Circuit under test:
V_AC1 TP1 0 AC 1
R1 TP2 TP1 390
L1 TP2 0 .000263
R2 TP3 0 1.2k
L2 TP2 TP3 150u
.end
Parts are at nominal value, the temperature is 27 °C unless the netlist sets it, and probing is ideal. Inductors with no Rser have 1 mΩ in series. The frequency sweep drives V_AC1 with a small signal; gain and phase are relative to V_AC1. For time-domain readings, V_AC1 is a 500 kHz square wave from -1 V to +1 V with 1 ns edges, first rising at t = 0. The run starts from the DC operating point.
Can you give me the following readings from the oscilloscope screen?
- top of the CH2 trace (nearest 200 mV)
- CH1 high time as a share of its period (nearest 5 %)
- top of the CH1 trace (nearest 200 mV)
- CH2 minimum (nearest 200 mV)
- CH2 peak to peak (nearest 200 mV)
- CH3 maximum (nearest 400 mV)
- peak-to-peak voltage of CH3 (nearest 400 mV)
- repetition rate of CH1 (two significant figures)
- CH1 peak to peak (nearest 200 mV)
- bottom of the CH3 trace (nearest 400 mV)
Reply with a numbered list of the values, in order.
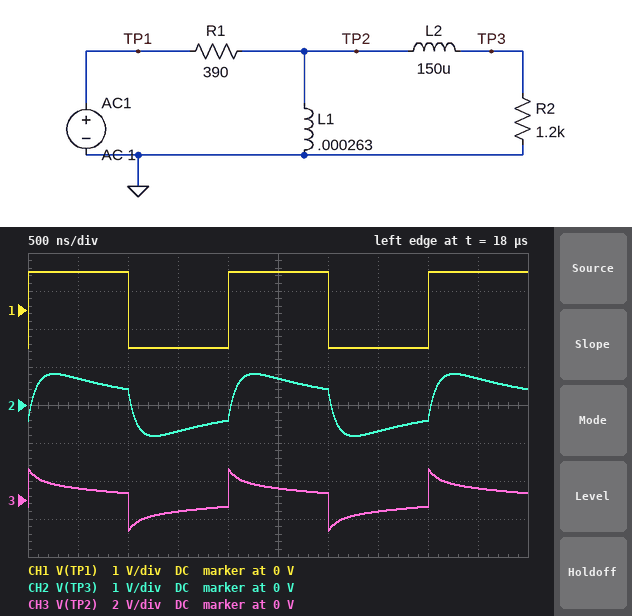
1. 800 mV
2. 50 %
3. 1.0 V
4. -800 mV
5. 1.6 V
6. 1.6 V
7. 3.2 V
8. 500 kHz
9. 2.0 V
10. -1.6 V
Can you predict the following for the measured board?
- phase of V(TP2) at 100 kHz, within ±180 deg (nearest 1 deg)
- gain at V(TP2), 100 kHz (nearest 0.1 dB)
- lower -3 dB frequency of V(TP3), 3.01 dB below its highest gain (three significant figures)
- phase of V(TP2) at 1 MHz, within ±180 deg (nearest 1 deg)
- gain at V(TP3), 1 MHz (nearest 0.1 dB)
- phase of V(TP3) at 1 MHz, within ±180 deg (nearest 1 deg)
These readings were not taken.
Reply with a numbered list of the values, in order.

1. 61 deg
2. -8.7 dB
3. 145 kHz
4. 18 deg
5. -4.1 dB
6. -20 deg
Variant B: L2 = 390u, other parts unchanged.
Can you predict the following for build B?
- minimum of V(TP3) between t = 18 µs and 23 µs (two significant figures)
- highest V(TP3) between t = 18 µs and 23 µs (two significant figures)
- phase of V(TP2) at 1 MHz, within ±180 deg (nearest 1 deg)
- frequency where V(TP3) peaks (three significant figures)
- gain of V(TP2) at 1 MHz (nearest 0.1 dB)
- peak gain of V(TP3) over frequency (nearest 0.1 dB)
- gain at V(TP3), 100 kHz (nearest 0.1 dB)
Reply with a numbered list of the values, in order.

1. -590 mV
2. 590 mV
3. 19 deg
4. 340 kHz
5. -1.0 dB
6. -5.1 dB
7. -9.0 dB
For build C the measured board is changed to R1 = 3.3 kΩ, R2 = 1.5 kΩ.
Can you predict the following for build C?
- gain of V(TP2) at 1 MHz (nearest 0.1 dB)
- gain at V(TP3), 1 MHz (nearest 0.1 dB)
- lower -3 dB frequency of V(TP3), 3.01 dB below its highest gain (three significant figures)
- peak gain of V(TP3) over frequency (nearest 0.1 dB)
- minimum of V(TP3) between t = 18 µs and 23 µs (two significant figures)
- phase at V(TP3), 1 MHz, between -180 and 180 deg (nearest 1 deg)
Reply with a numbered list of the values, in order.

1. -11.9 dB
2. -13.4 dB
3. 423 kHz
4. -13.0 dB
5. -370 mV
6. 17 deg
